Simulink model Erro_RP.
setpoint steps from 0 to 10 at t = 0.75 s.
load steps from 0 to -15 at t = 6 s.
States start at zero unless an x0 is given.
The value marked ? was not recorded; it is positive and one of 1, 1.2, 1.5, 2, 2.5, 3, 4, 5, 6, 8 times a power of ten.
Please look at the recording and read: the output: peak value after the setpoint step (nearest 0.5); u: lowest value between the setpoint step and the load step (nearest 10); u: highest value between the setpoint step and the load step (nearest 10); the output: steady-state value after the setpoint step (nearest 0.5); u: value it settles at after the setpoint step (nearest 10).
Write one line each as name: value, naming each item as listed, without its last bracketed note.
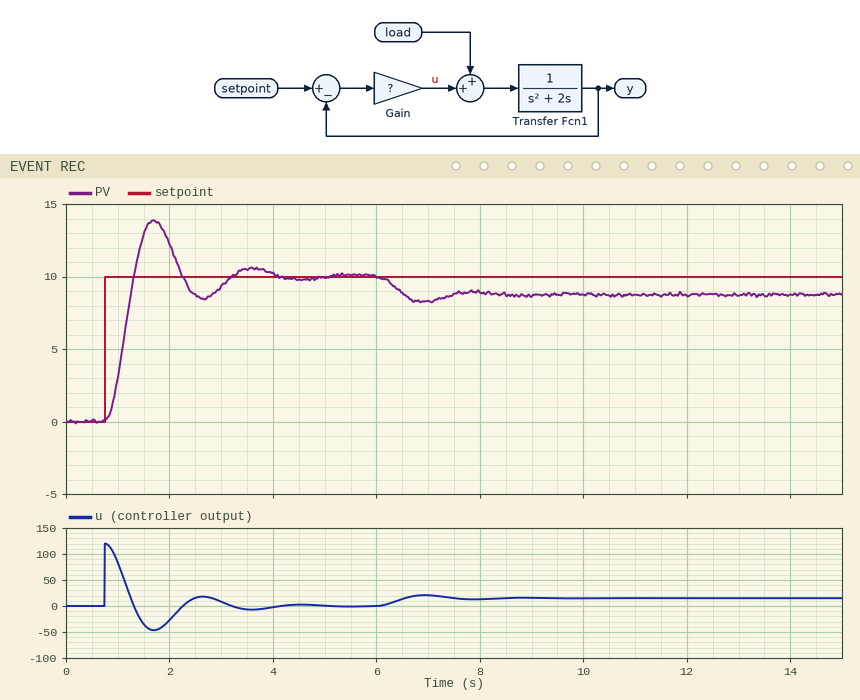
the output: peak value after the setpoint step: 14.0
u: lowest value between the setpoint step and the load step: -50
u: highest value between the setpoint step and the load step: 120
the output: steady-state value after the setpoint step: 10.0
u: value it settles at after the setpoint step: 0
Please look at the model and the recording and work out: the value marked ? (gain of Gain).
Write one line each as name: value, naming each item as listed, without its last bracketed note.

the value marked ?: 12
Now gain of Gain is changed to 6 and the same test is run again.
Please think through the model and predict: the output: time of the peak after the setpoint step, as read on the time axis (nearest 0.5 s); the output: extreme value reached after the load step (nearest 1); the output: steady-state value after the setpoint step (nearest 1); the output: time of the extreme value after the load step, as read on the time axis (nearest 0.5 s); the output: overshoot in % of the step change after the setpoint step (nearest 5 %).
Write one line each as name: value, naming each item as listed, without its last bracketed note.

the output: time of the peak after the setpoint step, as read on the time axis: 2.0 s
the output: extreme value reached after the load step: 7
the output: steady-state value after the setpoint step: 10
the output: time of the extreme value after the load step, as read on the time axis: 7.5 s
the output: overshoot in % of the step change after the setpoint step: 25 %
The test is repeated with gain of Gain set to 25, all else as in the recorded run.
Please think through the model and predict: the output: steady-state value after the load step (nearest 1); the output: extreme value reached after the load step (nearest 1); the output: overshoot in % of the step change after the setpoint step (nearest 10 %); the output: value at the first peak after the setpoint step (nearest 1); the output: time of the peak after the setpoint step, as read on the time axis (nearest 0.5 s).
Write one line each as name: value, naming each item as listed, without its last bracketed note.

the output: steady-state value after the load step: 9
the output: extreme value reached after the load step: 9
the output: overshoot in % of the step change after the setpoint step: 50 %
the output: value at the first peak after the setpoint step: 15
the output: time of the peak after the setpoint step, as read on the time axis: 1.5 s
